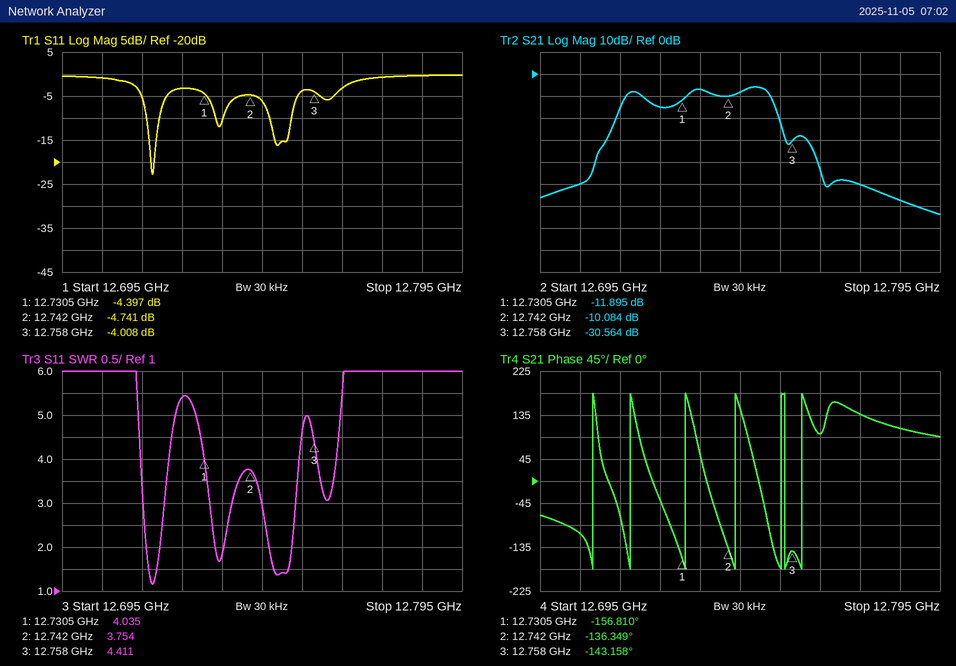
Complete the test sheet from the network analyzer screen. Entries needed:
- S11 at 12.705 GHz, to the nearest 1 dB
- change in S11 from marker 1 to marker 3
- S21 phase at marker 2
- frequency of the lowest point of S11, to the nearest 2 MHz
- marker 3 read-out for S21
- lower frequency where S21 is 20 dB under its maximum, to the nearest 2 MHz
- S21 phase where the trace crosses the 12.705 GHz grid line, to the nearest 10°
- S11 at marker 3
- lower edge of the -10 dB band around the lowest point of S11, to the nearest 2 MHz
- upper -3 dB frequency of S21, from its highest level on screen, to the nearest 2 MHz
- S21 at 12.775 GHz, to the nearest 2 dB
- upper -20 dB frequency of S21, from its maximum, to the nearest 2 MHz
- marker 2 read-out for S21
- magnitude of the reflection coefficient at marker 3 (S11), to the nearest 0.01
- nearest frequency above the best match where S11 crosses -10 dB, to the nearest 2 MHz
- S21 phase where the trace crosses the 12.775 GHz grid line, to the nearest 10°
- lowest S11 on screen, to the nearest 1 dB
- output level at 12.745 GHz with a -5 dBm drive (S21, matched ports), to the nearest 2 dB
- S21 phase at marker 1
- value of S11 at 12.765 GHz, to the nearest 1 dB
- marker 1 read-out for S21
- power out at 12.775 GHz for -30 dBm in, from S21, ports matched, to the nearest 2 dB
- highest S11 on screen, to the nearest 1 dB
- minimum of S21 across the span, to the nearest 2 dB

-1 dB
0.389 dB
-136.349°
12.718 GHz
-30.564 dB
12.712 GHz
-110°
-4.008 dB
12.716 GHz
12.752 GHz
-50 dB
12.756 GHz
-10.084 dB
0.63
12.720 GHz
140°
-23 dB
-14 dBm
-156.810°
-3 dB
-11.895 dB
-80 dBm
0 dB
-64 dB
